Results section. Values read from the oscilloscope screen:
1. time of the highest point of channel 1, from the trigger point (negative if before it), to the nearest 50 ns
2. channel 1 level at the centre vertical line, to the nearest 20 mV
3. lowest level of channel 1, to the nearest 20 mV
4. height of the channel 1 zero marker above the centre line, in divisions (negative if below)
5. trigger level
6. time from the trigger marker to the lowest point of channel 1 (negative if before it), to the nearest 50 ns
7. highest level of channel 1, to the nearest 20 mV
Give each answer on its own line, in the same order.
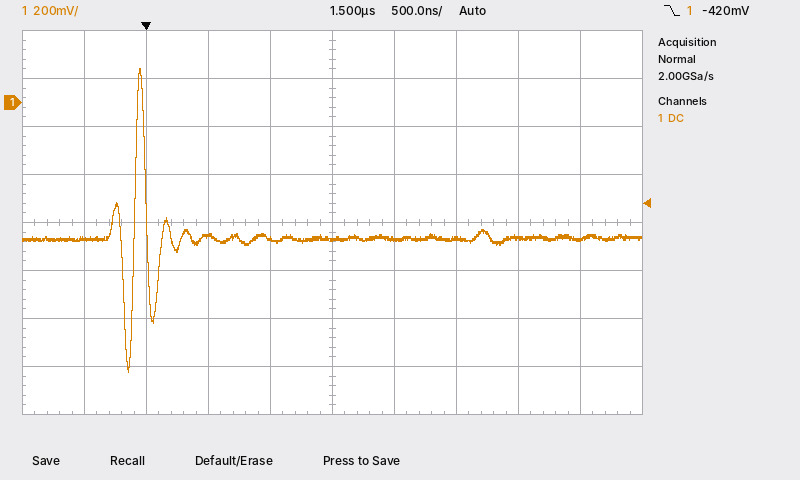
-50 ns
-580 mV
-1.12 V
+2.5 div
-420 mV
-150 ns
140 mV
